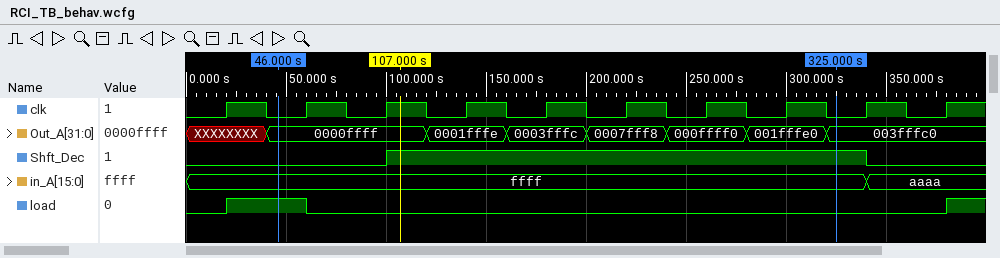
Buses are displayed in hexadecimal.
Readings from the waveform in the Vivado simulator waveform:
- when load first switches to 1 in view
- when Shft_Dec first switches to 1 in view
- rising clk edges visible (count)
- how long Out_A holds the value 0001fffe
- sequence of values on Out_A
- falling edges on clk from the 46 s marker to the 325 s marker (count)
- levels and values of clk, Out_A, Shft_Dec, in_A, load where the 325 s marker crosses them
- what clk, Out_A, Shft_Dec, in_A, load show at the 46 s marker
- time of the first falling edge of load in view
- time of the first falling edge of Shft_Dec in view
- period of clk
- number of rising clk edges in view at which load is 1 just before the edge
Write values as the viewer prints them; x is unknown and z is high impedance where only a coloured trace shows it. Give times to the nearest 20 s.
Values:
20 s
100 s
10
40 s
XXXXXXXX, 0000ffff, 0001fffe, 0003fffc, 0007fff8, 000ffff0, 001fffe0, 003fffc0
7
clk=0, Out_A=003fffc0, Shft_Dec=1, in_A=ffff, load=0
clk=0, Out_A=0000ffff, Shft_Dec=0, in_A=ffff, load=1
60 s
340 s
40 s
1
